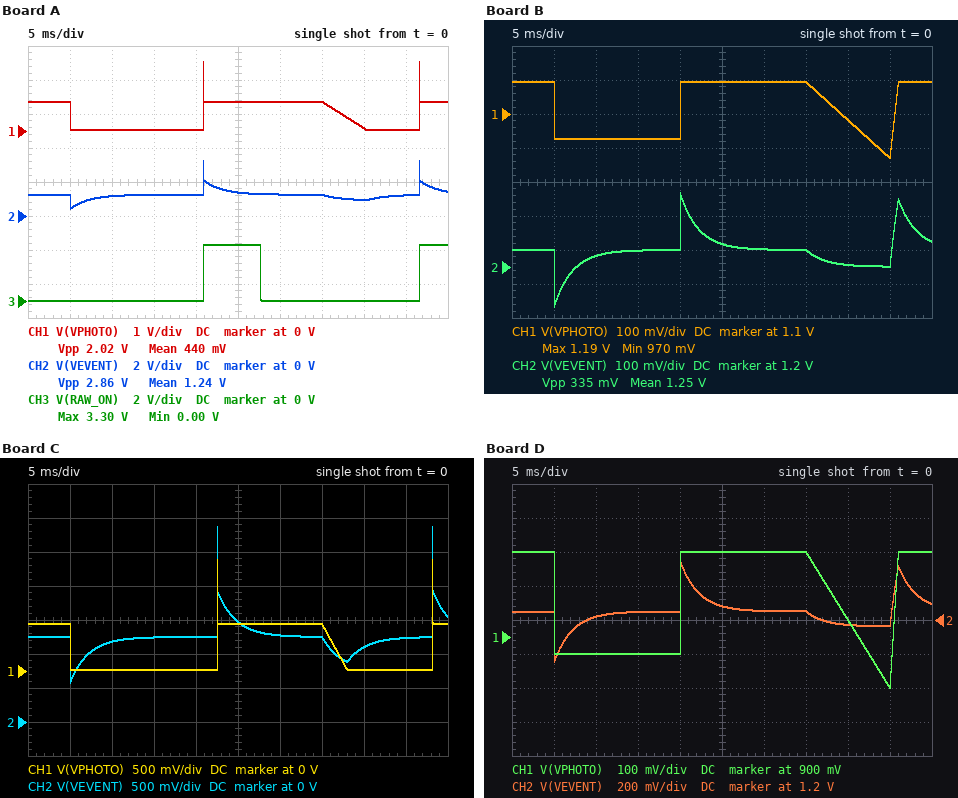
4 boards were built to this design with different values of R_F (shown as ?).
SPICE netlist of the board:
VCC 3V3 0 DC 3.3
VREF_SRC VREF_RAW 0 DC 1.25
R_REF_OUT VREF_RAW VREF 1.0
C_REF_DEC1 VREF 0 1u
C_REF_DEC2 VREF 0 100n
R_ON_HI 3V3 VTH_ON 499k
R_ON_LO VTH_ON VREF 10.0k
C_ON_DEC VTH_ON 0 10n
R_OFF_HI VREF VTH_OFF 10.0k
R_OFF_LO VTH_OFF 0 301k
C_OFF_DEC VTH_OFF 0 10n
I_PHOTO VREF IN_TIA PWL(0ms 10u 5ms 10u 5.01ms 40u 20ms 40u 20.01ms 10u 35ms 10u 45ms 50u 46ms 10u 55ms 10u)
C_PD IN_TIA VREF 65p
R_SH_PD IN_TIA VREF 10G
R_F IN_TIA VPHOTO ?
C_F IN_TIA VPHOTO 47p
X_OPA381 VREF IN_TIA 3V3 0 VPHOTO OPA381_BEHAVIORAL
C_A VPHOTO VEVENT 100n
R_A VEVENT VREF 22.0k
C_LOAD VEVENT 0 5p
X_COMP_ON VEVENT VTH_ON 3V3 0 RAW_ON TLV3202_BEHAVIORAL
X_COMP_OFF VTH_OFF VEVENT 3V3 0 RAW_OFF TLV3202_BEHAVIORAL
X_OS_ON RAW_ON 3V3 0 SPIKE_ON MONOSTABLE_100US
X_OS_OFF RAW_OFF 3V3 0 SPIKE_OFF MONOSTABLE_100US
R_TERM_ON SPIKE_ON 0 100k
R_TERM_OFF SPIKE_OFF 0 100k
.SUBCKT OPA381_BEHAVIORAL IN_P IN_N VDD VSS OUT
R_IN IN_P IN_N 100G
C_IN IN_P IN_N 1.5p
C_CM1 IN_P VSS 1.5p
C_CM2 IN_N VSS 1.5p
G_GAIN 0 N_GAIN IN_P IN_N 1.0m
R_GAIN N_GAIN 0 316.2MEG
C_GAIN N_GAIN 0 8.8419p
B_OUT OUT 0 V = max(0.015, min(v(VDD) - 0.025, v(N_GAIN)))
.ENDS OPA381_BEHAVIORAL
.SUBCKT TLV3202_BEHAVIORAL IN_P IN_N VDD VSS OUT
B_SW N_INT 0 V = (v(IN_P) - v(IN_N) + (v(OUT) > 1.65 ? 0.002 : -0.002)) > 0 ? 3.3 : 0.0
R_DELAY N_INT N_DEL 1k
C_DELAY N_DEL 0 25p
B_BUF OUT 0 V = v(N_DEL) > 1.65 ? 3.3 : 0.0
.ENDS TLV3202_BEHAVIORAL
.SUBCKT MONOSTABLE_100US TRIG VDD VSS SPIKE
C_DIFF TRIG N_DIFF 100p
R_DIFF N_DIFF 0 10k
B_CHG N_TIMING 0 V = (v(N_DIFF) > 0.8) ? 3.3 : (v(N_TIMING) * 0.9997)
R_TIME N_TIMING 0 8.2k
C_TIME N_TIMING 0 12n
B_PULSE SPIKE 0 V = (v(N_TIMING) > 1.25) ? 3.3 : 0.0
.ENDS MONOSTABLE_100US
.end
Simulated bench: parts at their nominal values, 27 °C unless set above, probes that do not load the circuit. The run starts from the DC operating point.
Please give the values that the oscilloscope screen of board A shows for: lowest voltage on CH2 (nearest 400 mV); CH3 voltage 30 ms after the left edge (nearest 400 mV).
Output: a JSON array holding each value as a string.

["400 mV", "0 V"]
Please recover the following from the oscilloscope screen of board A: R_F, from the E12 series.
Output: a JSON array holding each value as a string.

["39 kΩ"]
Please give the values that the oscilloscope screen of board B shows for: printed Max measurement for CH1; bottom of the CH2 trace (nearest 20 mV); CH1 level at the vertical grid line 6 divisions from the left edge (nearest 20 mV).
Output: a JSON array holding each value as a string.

["1.19 V", "1.08 V", "1.20 V"]
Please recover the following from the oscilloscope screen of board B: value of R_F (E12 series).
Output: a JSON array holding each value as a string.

["5.6 kΩ"]
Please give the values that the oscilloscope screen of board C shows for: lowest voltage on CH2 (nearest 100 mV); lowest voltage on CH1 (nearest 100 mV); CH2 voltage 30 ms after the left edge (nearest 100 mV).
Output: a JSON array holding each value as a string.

["600 mV", "0 V", "1.3 V"]
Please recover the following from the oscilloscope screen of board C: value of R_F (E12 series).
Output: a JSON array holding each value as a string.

["56 kΩ"]
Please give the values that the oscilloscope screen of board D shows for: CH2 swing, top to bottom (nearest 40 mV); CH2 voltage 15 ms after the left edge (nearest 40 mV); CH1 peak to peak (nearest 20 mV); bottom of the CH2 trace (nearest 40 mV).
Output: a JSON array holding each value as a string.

["600 mV", "1.24 V", "400 mV", "960 mV"]
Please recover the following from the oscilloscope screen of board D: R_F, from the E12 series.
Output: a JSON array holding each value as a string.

["10 kΩ"]
